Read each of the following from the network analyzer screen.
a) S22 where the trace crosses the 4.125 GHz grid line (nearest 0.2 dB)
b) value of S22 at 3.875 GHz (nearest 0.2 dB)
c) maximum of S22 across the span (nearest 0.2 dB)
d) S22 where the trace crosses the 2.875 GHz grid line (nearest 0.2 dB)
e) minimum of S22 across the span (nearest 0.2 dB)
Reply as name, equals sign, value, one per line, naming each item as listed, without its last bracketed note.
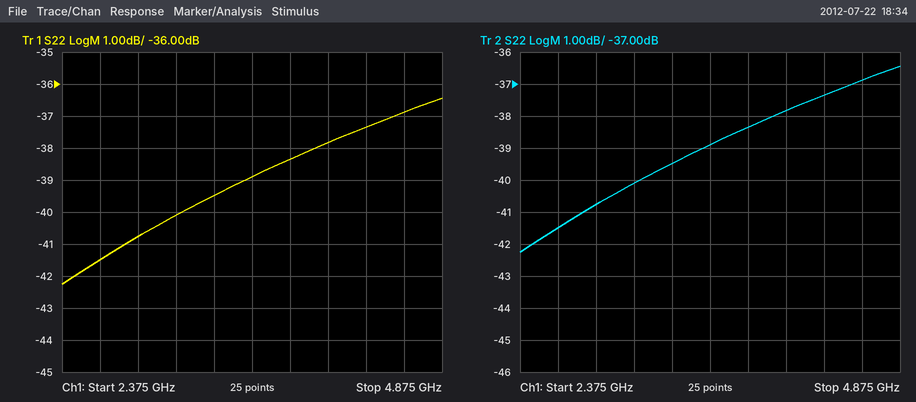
S22 where the trace crosses the 4.125 GHz grid line = -37.8 dB
value of S22 at 3.875 GHz = -38.4 dB
maximum of S22 across the span = -36.4 dB
S22 where the trace crosses the 2.875 GHz grid line = -40.8 dB
minimum of S22 across the span = -42.2 dB
